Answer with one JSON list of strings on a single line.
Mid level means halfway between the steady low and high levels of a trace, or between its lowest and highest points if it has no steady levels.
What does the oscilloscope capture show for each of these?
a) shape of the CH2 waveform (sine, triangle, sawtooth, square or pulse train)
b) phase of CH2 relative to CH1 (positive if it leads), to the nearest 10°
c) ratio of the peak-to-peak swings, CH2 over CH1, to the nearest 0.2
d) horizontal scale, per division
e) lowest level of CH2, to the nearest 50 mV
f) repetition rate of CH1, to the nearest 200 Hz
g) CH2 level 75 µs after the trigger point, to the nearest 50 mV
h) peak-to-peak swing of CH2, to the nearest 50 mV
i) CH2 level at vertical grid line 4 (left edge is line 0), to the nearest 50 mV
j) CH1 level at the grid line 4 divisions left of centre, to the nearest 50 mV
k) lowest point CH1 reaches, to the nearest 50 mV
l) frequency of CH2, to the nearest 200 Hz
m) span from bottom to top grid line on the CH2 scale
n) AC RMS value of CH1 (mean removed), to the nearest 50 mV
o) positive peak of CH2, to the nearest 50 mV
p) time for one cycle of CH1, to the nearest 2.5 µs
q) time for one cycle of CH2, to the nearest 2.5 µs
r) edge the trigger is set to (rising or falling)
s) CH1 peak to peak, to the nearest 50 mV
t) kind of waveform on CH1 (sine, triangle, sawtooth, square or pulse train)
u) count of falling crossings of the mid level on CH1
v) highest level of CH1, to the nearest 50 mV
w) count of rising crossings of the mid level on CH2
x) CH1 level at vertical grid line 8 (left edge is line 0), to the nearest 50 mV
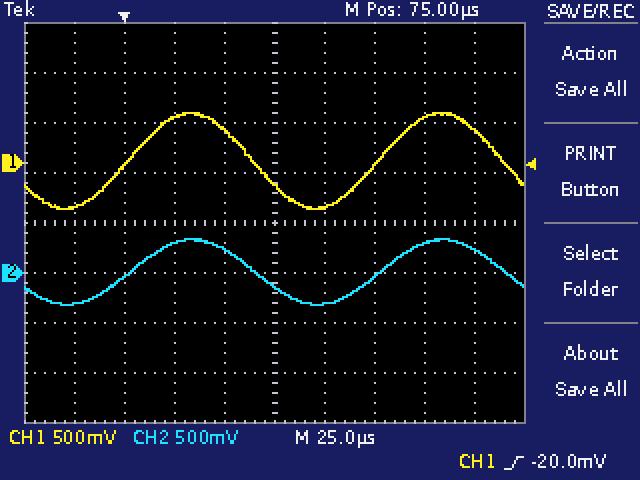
["sine", "0°", "0.6", "25 µs", "-300 mV", "8.0 kHz", "-150 mV", "650 mV", "250 mV", "-450 mV", "-450 mV", "8.0 kHz", "4 V", "350 mV", "350 mV", "125.0 µs", "125.0 µs", "rising", "950 mV", "sine", "2", "500 mV", "2", "450 mV"]
